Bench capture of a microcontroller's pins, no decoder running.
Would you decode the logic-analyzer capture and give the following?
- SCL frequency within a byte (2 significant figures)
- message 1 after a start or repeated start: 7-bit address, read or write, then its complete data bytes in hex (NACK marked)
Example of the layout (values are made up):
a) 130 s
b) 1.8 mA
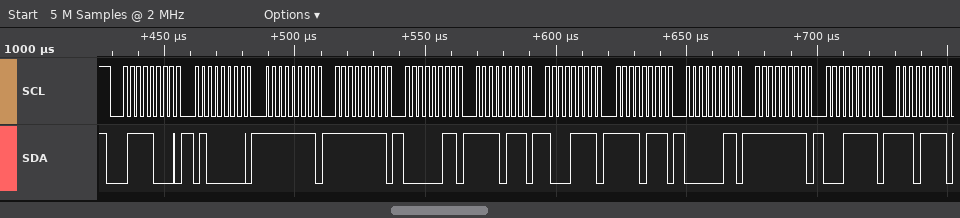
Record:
a) 400 kHz
b) 0x3C write: 40 FF FF 03 F7 8F F7 03 FF 1F EF
